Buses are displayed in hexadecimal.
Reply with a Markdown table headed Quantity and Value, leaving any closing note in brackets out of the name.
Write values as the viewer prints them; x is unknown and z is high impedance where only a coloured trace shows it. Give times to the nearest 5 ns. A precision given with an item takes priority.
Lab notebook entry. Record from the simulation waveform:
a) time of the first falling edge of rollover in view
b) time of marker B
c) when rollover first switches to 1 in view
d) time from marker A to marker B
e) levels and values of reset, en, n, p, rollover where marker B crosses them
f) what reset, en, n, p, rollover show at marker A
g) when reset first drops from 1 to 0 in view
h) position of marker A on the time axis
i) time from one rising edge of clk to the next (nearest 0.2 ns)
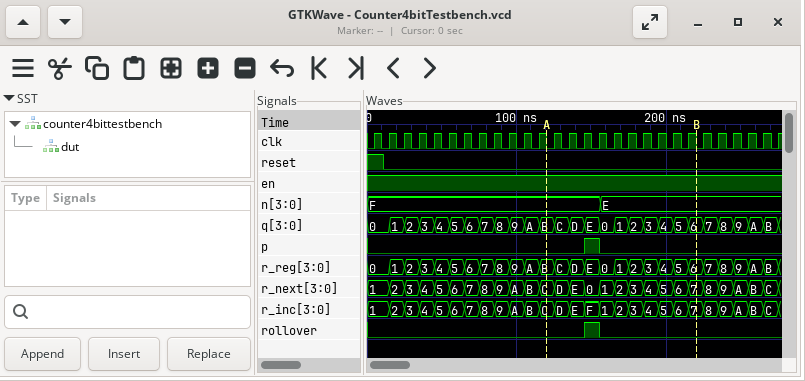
| Quantity | Value |
|---|---|
| time of the first falling edge of rollover in view | 155 ns |
| time of marker B | 220 ns |
| when rollover first switches to 1 in view | 145 ns |
| time from marker A to marker B | 100 ns |
| levels and values of reset, en, n, p, rollover where marker B crosses them | reset=0, en=1, n=E, p=0, rollover=0 |
| what reset, en, n, p, rollover show at marker A | reset=0, en=1, n=F, p=0, rollover=0 |
| when reset first drops from 1 to 0 in view | 10 ns |
| position of marker A on the time axis | 120 ns |
| time from one rising edge of clk to the next | 10 ns |
